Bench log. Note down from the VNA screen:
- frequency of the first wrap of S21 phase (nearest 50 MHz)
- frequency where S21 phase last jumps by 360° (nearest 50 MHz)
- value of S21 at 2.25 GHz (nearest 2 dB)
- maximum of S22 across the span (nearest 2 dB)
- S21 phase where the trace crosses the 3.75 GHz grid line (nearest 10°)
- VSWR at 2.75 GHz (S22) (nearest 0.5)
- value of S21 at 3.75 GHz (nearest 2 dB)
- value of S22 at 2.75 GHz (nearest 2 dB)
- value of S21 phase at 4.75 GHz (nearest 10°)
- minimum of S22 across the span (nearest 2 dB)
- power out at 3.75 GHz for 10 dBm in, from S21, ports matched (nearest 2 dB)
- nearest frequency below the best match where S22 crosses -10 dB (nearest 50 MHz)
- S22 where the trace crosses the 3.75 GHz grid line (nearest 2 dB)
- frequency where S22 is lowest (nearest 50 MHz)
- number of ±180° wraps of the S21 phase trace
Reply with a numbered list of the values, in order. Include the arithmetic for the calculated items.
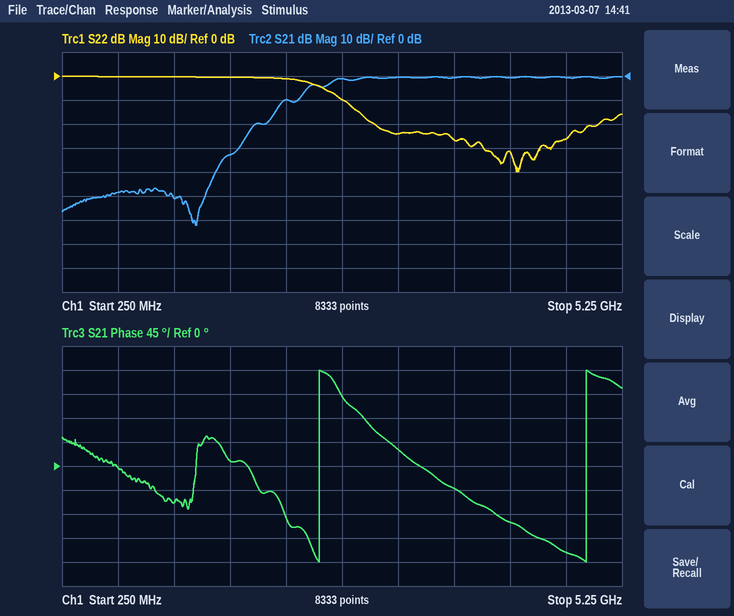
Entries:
1. 2.55 GHz
2. 4.95 GHz
3. -10 dB
4. 0 dB
5. -40°
6. |Γ| = 10^(-10/20) = 0.3162; VSWR = (1 + 0.3162)/(1 − 0.3162) ≈ 1.92, so 2.0 to the nearest 0.5
7. 0 dB
8. -10 dB
9. -160°
10. -40 dB
11. 10 dBm + (0 dB) = 10 dBm
12. 2.75 GHz
13. -26 dB
14. 4.30 GHz
15. 2
